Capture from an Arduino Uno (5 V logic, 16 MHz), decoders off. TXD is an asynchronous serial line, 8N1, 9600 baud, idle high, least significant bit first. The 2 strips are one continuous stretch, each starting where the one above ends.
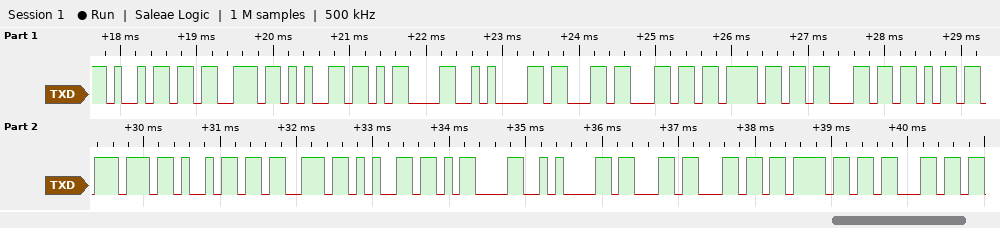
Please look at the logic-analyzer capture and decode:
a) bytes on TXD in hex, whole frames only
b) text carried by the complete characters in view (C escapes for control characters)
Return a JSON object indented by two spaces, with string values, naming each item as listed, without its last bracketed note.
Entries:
{
  "bytes on TXD in hex, whole frames only": "69 73 65 0D 0A 63 6C 6F 63 6B 77 69 73 65 0D 0A 63 6C 6F 63",
  "text carried by the complete characters in view": "\"ise\\r\\nclockwise\\r\\ncloc\""
}
